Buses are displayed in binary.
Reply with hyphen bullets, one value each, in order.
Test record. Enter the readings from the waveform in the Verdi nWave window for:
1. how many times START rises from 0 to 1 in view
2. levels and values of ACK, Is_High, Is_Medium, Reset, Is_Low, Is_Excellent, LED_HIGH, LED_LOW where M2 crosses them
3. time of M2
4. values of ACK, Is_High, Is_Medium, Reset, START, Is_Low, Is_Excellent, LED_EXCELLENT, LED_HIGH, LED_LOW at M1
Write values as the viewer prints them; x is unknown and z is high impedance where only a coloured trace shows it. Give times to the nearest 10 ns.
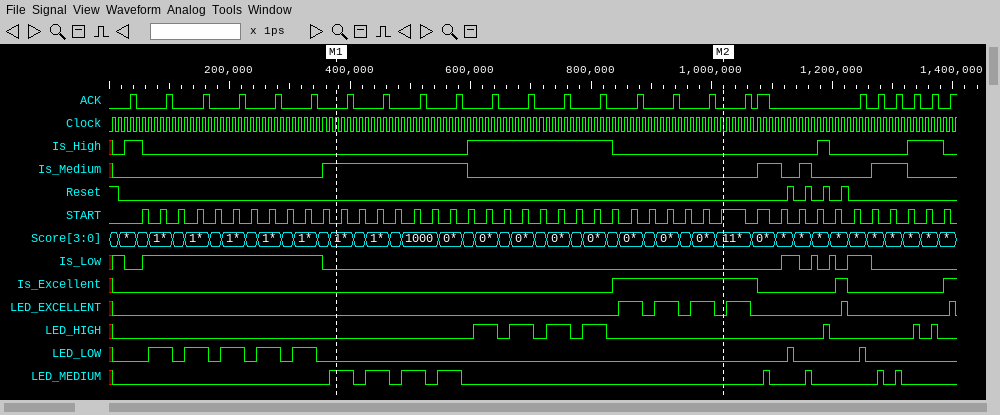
- 44
- ACK=0, Is_High=0, Is_Medium=0, Reset=0, Is_Low=0, Is_Excellent=1, LED_HIGH=0, LED_LOW=0
- 1020 ns
- ACK=0, Is_High=0, Is_Medium=1, Reset=0, START=0, Is_Low=0, Is_Excellent=0, LED_EXCELLENT=0, LED_HIGH=0, LED_LOW=0
